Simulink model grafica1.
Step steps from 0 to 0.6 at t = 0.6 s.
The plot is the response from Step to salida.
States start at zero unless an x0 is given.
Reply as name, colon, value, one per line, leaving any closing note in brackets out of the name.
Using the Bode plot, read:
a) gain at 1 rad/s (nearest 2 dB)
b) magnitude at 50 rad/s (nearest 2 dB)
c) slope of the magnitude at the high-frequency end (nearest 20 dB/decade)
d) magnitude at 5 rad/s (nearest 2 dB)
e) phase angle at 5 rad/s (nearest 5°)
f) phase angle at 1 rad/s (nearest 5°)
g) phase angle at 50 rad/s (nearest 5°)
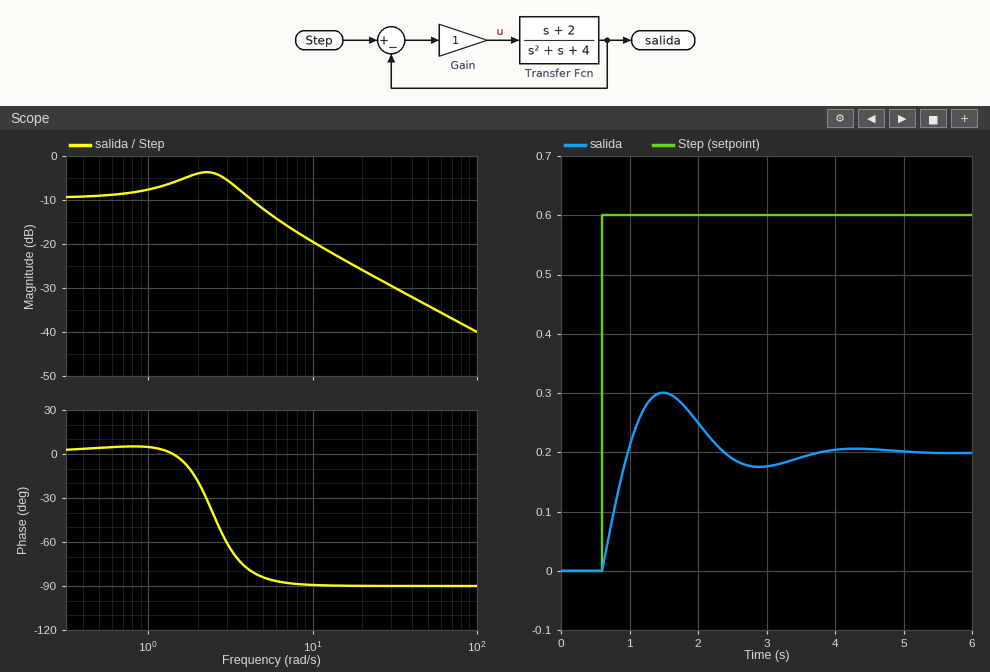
gain at 1 rad/s: -8 dB
magnitude at 50 rad/s: -34 dB
slope of the magnitude at the high-frequency end: -20 dB/decade
magnitude at 5 rad/s: -12 dB
phase angle at 5 rad/s: -85°
phase angle at 1 rad/s: 5°
phase angle at 50 rad/s: -90°
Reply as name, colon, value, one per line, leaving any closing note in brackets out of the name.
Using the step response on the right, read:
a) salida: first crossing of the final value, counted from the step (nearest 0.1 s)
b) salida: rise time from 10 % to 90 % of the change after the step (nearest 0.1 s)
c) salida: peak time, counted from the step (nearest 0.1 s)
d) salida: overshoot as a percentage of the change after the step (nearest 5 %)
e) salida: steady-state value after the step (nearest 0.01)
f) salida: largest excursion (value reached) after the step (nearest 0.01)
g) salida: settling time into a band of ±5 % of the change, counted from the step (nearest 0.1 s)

salida: first crossing of the final value, counted from the step: 0.4 s
salida: rise time from 10 % to 90 % of the change after the step: 0.3 s
salida: peak time, counted from the step: 0.9 s
salida: overshoot as a percentage of the change after the step: 50 %
salida: steady-state value after the step: 0.20
salida: largest excursion (value reached) after the step: 0.30
salida: settling time into a band of ±5 % of the change, counted from the step: 2.9 s
